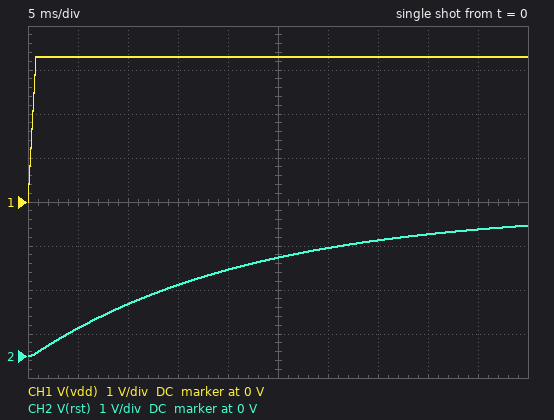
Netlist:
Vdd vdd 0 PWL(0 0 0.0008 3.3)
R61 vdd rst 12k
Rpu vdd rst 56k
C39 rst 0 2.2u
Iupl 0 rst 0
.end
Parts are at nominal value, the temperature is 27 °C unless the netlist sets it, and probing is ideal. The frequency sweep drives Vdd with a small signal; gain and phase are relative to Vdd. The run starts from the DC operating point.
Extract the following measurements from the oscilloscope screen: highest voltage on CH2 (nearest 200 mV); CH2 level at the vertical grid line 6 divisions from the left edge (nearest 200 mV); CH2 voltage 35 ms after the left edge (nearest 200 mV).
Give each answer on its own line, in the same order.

3.0 V
2.4 V
2.6 V
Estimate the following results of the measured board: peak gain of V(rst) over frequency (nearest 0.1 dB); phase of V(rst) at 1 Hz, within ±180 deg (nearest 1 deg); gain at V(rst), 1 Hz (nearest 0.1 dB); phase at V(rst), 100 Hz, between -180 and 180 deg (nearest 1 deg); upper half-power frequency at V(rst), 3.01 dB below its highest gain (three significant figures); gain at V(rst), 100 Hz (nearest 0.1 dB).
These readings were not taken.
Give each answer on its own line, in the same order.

0 dB
-8 deg
-0.1 dB
-86 deg
7.32 Hz
-22.7 dB
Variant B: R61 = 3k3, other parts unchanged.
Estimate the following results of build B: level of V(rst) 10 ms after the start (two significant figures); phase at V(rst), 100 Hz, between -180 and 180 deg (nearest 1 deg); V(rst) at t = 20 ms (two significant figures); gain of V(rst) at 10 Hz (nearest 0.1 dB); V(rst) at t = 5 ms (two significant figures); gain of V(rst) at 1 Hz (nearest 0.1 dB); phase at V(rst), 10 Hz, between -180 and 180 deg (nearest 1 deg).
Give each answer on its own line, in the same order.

2.5 V
-77 deg
3.1 V
-0.7 dB
1.6 V
0 dB
-23 deg
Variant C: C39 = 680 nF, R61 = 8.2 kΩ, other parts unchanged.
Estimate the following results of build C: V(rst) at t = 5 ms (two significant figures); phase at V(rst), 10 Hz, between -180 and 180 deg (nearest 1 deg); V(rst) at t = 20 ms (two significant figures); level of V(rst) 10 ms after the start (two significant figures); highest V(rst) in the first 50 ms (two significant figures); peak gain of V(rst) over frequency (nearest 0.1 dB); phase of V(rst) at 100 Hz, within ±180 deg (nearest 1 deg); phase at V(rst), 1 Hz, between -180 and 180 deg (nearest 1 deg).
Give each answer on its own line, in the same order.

2.0 V
-17 deg
3.2 V
2.8 V
3.3 V
0 dB
-72 deg
-2 deg
